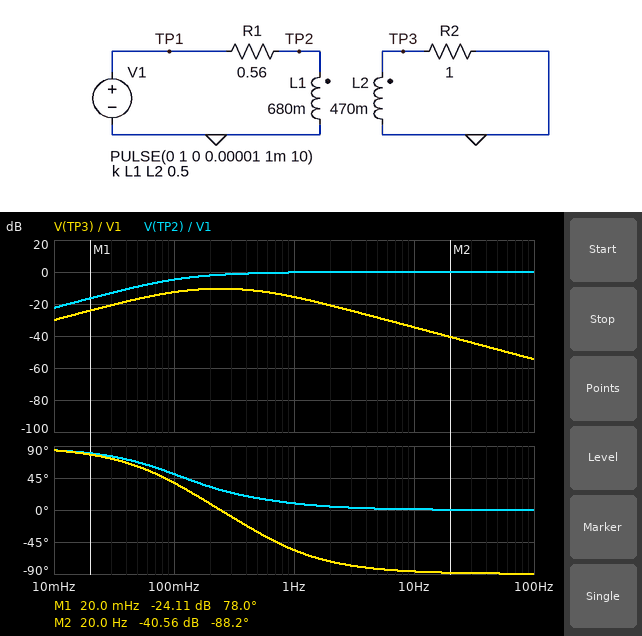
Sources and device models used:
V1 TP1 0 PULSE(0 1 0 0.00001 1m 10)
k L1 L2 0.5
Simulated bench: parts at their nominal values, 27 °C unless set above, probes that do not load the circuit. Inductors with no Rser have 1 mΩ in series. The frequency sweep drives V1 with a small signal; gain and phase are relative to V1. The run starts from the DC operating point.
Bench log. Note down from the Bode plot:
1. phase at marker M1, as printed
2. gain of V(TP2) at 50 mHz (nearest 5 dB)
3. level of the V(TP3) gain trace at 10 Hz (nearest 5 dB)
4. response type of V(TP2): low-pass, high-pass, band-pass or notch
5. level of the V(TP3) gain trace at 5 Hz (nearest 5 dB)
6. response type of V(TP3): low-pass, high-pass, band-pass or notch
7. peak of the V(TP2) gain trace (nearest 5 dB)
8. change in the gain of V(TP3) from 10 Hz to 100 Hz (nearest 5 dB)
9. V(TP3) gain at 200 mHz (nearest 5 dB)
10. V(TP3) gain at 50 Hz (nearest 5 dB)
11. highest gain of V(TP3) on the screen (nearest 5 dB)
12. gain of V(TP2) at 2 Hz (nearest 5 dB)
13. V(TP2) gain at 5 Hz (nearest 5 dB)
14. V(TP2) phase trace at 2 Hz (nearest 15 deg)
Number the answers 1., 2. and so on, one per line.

1. 78.0 deg
2. -10 dB
3. -35 dB
4. high-pass
5. -30 dB
6. band-pass
7. 0 dB
8. -20 dB
9. -10 dB
10. -50 dB
11. -10 dB
12. 0 dB
13. 0 dB
14. 0 deg
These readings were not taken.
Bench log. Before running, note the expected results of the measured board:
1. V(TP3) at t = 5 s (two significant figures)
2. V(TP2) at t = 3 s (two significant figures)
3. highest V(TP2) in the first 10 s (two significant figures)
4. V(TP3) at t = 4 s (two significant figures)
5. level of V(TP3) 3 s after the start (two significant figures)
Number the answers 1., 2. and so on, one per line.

1. 12 mV
2. 97 mV
3. 1.0 V
4. 26 mV
5. 53 mV
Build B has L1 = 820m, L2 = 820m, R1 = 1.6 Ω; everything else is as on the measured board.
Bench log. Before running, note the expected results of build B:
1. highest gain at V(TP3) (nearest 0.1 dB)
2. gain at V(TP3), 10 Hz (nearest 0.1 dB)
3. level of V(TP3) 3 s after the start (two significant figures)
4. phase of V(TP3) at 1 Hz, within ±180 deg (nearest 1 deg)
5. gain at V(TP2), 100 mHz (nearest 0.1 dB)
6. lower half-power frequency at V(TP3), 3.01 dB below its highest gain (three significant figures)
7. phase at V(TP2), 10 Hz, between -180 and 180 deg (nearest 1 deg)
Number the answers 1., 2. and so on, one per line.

1. -14.3 dB
2. -37.8 dB
3. 19 mV
4. -54 deg
5. -10.9 dB
6. 104 mHz
7. 2 deg
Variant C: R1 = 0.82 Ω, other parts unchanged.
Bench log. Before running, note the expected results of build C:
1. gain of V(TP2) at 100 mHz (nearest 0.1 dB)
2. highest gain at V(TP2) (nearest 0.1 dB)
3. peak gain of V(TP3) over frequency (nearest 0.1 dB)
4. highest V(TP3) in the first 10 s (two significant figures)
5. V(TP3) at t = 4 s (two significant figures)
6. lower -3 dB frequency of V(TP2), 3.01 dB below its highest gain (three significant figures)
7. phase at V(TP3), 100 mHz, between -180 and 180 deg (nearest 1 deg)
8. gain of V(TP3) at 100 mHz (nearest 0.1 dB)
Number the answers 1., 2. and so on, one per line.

1. -7.1 dB
2. 0 dB
3. -11.5 dB
4. 210 mV
5. 9.1 mV
6. 235 mHz
7. 47 deg
8. -14.9 dB
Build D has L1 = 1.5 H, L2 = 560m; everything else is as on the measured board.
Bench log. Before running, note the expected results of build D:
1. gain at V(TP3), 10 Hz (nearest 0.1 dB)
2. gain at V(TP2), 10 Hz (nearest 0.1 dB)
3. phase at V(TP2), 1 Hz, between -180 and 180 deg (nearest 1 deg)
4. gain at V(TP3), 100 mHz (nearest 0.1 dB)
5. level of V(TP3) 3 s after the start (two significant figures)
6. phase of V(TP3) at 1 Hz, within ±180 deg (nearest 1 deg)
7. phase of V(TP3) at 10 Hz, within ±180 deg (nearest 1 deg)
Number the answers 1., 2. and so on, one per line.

1. -38.7 dB
2. 0 dB
3. 4 deg
4. -12.3 dB
5. 120 mV
6. -65 deg
7. -87 deg
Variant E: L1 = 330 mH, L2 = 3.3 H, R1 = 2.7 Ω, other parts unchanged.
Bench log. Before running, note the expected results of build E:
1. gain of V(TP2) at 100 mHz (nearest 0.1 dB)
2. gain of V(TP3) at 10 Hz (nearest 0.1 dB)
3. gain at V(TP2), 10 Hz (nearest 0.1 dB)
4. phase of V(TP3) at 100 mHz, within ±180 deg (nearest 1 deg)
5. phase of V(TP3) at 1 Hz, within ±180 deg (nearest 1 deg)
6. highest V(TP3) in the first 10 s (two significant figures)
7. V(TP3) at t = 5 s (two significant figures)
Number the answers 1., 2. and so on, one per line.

1. -24.3 dB
2. -40.0 dB
3. -0.1 dB
4. 22 deg
5. -27 deg
6. 52 mV
7. 13 mV
